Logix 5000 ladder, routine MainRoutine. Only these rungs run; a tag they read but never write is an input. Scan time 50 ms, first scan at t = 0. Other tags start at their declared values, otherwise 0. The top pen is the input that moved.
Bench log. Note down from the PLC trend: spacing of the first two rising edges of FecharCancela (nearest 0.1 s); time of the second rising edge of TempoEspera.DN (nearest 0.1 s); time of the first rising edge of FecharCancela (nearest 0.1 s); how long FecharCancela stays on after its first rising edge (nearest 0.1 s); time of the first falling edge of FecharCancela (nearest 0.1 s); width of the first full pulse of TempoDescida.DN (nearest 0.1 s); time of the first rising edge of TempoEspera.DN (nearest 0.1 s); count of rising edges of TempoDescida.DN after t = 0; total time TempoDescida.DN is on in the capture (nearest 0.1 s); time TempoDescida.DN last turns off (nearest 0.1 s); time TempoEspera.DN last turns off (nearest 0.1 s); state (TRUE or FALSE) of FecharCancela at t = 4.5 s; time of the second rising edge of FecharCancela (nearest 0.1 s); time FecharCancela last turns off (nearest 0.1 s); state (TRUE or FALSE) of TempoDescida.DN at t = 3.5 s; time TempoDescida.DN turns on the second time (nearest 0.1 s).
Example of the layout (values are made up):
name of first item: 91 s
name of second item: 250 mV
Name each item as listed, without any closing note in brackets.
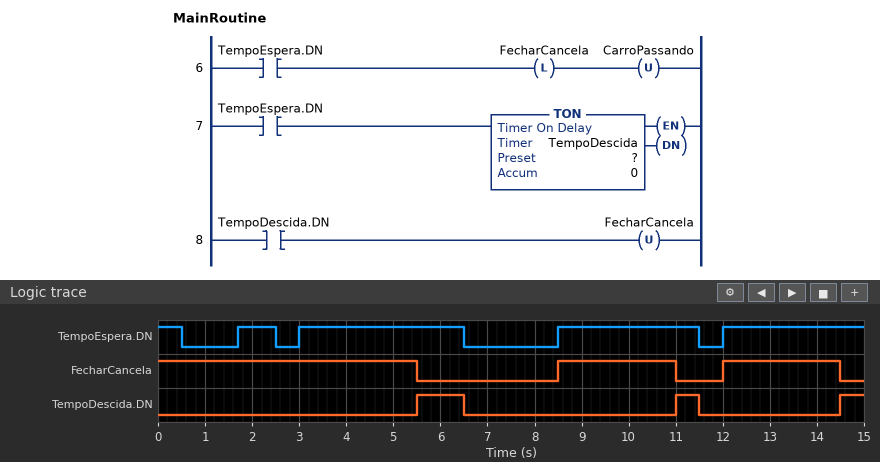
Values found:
spacing of the first two rising edges of FecharCancela: 3.5 s
time of the second rising edge of TempoEspera.DN: 3.0 s
time of the first rising edge of FecharCancela: 8.5 s
how long FecharCancela stays on after its first rising edge: 2.5 s
time of the first falling edge of FecharCancela: 5.5 s
width of the first full pulse of TempoDescida.DN: 1.0 s
time of the first rising edge of TempoEspera.DN: 1.7 s
count of rising edges of TempoDescida.DN after t = 0: 3
total time TempoDescida.DN is on in the capture: 2.0 s
time TempoDescida.DN last turns off: 11.5 s
time TempoEspera.DN last turns off: 11.5 s
state (TRUE or FALSE) of FecharCancela at t = 4.5 s: TRUE
time of the second rising edge of FecharCancela: 12.0 s
time FecharCancela last turns off: 14.5 s
state (TRUE or FALSE) of TempoDescida.DN at t = 3.5 s: FALSE
time TempoDescida.DN turns on the second time: 11.0 s
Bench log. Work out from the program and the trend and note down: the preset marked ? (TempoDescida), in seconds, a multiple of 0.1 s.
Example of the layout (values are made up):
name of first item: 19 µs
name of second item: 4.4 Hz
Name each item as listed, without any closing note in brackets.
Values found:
the preset marked ? (TempoDescida), in seconds, a multiple of 0.1 s: 2.5 s
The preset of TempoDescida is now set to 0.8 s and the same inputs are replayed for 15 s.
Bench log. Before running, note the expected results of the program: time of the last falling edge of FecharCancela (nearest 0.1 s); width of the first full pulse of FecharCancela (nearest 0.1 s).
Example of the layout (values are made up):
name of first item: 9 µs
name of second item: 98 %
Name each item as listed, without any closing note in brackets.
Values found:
time of the last falling edge of FecharCancela: 12.8 s
width of the first full pulse of FecharCancela: 0.8 s
